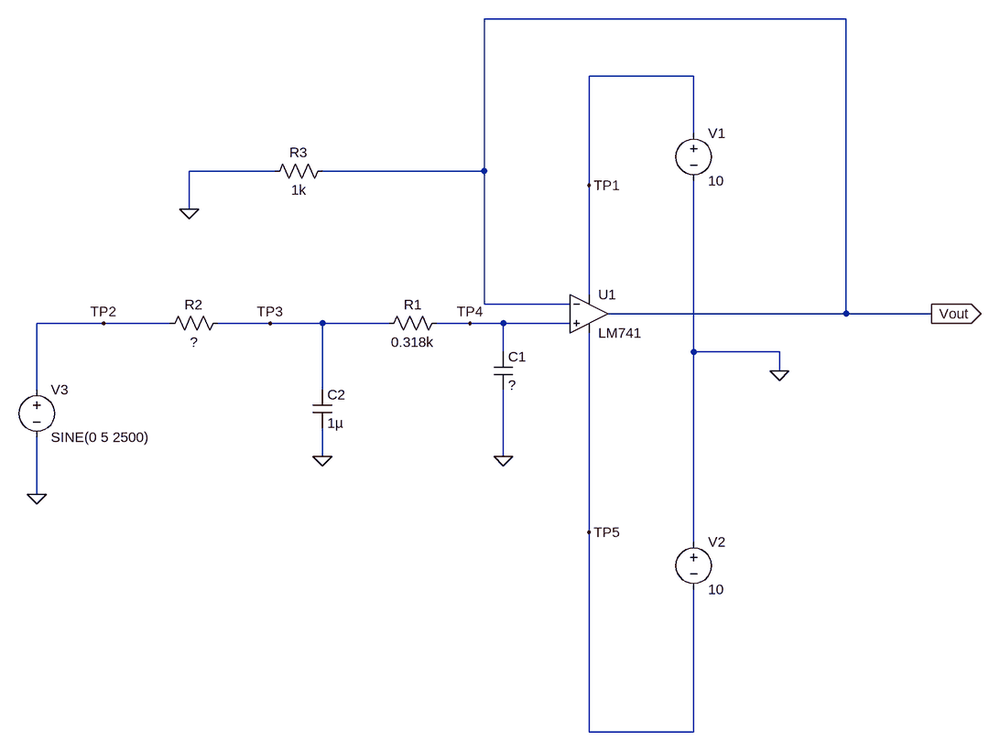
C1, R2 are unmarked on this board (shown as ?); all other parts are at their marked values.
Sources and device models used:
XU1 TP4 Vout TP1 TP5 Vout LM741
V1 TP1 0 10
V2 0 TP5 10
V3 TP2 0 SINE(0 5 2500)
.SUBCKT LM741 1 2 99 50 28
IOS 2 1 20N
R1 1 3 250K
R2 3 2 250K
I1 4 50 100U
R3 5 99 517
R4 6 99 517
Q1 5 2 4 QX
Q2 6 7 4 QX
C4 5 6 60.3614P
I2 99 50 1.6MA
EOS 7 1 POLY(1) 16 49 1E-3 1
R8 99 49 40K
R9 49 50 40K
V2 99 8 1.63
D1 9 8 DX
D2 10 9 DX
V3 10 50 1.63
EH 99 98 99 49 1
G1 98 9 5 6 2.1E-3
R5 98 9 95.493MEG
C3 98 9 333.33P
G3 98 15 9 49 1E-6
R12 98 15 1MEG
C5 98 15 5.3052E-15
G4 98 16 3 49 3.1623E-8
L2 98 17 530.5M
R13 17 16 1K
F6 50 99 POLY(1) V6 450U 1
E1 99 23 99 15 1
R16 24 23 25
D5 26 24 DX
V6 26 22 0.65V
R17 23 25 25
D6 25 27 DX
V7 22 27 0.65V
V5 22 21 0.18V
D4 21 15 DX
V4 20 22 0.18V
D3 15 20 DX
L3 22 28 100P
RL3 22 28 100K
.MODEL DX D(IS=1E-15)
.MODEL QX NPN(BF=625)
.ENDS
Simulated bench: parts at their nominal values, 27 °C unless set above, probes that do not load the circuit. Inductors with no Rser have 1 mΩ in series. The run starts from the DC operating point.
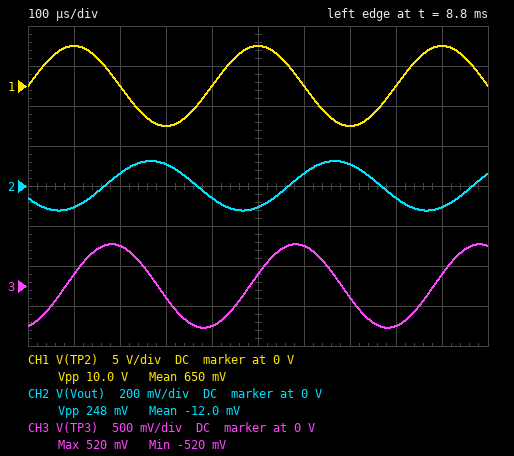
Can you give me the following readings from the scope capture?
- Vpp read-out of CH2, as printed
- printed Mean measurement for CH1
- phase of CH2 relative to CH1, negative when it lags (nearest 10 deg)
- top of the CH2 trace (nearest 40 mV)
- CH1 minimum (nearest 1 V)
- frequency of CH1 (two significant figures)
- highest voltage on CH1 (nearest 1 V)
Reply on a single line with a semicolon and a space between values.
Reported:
248 mV; 650 mV; -150 deg; 120 mV; -5 V; 2.5 kHz; 5 V
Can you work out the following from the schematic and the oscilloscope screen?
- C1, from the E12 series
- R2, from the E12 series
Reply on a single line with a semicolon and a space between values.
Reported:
820 nF; 560 Ω
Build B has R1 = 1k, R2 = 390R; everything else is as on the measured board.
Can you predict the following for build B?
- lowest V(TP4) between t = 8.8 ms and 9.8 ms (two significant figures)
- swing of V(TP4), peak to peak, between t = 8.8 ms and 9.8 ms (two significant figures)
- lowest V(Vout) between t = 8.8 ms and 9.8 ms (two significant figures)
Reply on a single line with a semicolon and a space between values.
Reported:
-61 mV; 120 mV; -60 mV
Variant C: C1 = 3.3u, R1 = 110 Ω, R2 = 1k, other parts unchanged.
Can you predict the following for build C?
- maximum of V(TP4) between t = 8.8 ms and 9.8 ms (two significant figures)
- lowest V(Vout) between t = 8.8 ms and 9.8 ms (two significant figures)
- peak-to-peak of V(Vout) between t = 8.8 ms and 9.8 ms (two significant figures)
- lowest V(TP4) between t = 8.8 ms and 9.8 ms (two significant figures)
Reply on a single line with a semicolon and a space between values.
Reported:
53 mV; -34 mV; 88 mV; -35 mV
